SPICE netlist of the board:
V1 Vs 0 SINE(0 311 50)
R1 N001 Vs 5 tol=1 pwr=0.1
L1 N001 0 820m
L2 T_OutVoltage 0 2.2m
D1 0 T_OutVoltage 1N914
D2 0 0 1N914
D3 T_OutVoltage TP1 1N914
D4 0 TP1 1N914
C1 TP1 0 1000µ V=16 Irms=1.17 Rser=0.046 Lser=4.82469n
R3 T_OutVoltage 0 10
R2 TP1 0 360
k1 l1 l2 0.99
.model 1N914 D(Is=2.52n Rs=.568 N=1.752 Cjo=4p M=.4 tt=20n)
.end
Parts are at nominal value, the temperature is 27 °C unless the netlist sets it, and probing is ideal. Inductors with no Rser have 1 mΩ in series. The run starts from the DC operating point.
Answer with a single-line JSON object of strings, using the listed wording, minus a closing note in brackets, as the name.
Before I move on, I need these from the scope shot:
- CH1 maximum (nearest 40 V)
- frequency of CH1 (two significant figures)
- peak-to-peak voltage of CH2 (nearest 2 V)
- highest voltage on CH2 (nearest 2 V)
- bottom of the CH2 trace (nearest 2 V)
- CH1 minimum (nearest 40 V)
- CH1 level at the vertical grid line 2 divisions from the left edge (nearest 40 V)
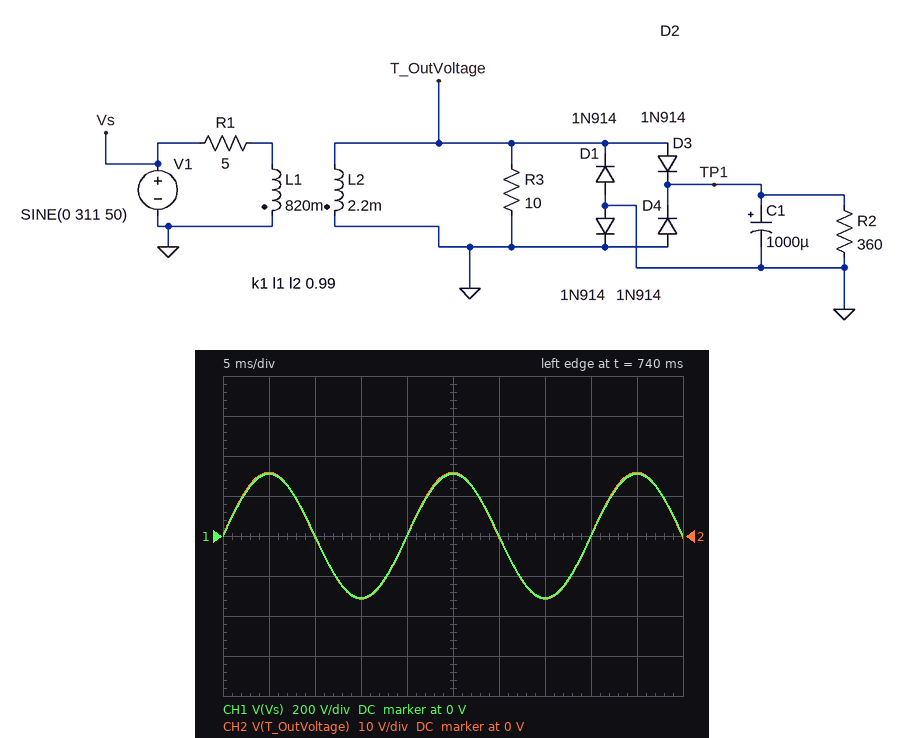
{"CH1 maximum": "320 V", "frequency of CH1": "50 Hz", "peak-to-peak voltage of CH2": "32 V", "highest voltage on CH2": "16 V", "bottom of the CH2 trace": "-16 V", "CH1 minimum": "-320 V", "CH1 level at the vertical grid line 2 divisions from the left edge": "0 V"}
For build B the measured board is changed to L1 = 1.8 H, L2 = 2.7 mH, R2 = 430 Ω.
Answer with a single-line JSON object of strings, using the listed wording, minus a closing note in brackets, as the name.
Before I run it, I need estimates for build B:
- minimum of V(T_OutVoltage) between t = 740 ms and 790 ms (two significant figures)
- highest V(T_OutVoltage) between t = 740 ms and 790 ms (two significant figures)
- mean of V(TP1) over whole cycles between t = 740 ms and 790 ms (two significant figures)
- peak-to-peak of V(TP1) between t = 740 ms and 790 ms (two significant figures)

{"minimum of V(T_OutVoltage) between t = 740 ms and 790 ms": "-12 V", "highest V(T_OutVoltage) between t = 740 ms and 790 ms": "12 V", "mean of V(TP1) over whole cycles between t = 740 ms and 790 ms": "11 V", "peak-to-peak of V(TP1) between t = 740 ms and 790 ms": "450 mV"}
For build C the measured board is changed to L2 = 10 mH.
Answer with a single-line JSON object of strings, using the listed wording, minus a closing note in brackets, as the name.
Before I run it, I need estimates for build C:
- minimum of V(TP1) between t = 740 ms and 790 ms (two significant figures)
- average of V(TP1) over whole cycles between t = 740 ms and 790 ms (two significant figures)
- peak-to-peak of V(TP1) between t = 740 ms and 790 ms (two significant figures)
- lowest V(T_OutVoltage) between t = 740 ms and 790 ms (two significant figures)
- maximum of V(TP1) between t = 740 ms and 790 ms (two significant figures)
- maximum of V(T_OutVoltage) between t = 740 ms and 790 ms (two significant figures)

{"minimum of V(TP1) between t = 740 ms and 790 ms": "30 V", "average of V(TP1) over whole cycles between t = 740 ms and 790 ms": "31 V", "peak-to-peak of V(TP1) between t = 740 ms and 790 ms": "1.6 V", "lowest V(T_OutVoltage) between t = 740 ms and 790 ms": "-31 V", "maximum of V(TP1) between t = 740 ms and 790 ms": "32 V", "maximum of V(T_OutVoltage) between t = 740 ms and 790 ms": "33 V"}
